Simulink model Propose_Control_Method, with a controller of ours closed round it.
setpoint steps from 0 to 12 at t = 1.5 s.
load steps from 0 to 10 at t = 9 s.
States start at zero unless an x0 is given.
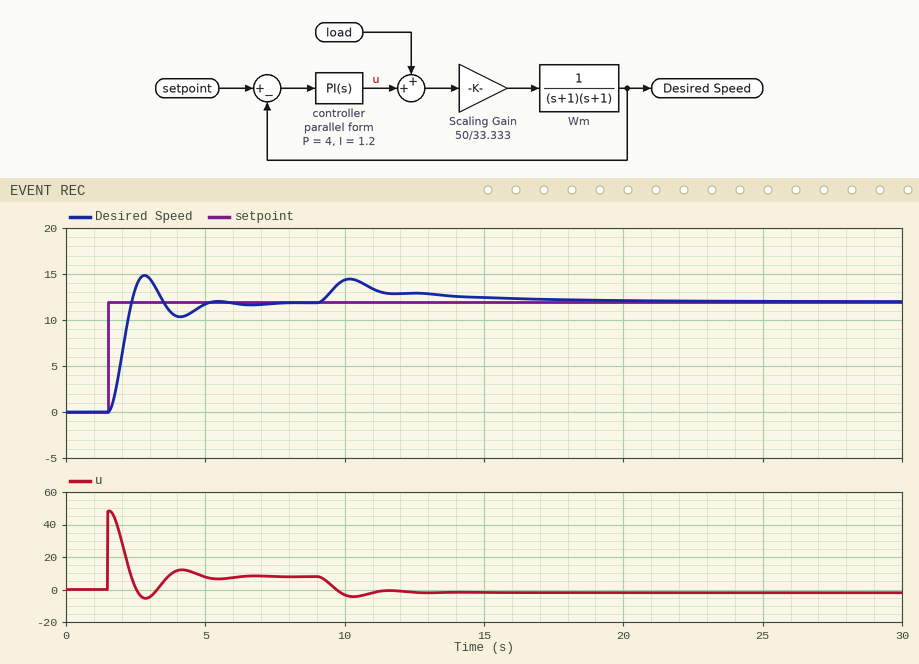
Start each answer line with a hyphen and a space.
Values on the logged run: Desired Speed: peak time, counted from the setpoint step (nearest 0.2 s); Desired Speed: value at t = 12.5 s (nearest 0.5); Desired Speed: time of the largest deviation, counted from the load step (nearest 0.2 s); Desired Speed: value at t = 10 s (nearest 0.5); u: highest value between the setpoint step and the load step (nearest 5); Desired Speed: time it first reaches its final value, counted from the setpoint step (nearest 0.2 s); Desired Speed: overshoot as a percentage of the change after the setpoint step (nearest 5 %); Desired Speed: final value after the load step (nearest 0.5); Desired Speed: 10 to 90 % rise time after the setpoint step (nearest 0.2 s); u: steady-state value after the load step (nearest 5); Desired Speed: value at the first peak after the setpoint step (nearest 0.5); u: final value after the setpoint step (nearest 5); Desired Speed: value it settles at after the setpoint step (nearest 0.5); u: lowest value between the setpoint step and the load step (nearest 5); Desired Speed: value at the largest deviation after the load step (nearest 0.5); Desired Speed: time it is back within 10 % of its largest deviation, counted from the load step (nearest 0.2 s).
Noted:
- 1.4 s
- 13.0
- 1.2 s
- 14.5
- 50
- 0.8 s
- 25 %
- 12.0
- 0.6 s
- 0
- 15.0
- 10
- 12.0
- -5
- 14.5
- 8.0 s
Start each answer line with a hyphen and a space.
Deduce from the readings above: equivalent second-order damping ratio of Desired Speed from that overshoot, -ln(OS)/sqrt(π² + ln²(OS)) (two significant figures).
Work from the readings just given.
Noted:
- 0.40
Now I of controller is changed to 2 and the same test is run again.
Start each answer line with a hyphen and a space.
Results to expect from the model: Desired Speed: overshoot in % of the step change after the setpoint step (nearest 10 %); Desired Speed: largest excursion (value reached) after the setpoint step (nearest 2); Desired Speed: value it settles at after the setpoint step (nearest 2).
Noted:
- 30 %
- 16
- 12
